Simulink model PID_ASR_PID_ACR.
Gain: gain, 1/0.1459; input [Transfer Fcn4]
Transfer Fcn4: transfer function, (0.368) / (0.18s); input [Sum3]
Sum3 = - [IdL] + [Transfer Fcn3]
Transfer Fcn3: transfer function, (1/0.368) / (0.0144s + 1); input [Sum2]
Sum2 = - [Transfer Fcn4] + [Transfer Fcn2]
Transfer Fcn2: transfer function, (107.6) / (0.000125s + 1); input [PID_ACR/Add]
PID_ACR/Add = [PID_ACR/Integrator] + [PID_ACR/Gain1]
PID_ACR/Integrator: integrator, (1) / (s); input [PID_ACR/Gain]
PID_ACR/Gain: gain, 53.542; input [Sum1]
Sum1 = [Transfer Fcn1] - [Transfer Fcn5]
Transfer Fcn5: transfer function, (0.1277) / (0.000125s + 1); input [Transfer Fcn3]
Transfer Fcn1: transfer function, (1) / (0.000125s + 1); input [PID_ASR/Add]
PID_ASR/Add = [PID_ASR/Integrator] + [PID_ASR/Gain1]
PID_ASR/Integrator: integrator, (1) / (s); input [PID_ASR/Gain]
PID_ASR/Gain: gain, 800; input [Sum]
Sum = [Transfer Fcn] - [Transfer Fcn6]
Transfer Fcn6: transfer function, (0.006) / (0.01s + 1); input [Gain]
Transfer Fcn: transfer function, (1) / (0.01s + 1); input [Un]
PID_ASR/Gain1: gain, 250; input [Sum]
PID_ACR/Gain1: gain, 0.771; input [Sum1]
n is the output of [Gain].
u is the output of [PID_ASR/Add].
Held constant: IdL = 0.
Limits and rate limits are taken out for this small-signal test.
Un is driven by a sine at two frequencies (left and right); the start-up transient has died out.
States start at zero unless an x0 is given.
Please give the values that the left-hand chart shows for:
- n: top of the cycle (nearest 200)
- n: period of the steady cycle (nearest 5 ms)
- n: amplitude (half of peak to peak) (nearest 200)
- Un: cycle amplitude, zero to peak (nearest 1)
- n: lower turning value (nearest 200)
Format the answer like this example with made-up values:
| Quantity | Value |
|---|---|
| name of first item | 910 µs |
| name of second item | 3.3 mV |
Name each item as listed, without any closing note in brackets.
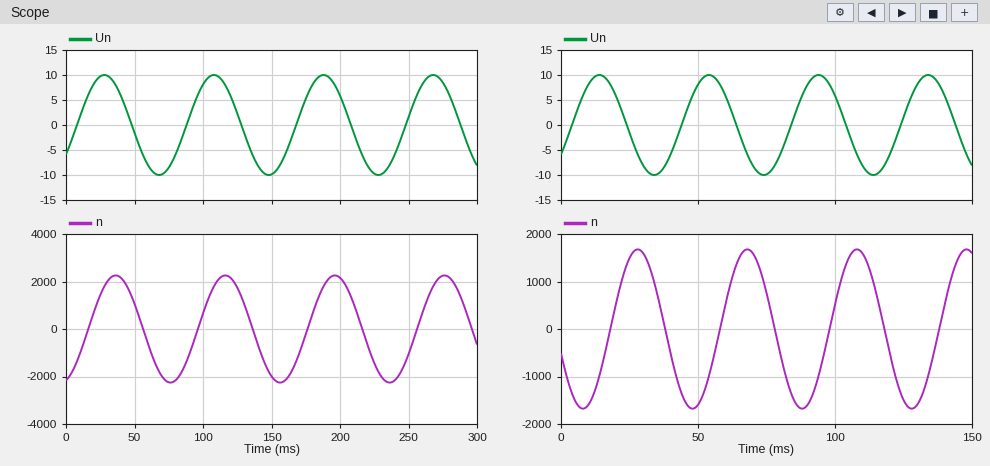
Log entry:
| Quantity | Value |
|---|---|
| n: top of the cycle | 2200 |
| n: period of the steady cycle | 80 ms |
| n: amplitude (half of peak to peak) | 2200 |
| Un: cycle amplitude, zero to peak | 10 |
| n: lower turning value | -2200 |
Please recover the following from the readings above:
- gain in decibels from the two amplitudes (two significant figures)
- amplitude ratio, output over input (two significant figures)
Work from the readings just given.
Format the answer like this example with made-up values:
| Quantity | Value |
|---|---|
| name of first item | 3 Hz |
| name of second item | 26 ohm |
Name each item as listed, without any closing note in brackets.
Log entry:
| Quantity | Value |
|---|---|
| gain in decibels from the two amplitudes | 47 dB |
| amplitude ratio, output over input | 220 |
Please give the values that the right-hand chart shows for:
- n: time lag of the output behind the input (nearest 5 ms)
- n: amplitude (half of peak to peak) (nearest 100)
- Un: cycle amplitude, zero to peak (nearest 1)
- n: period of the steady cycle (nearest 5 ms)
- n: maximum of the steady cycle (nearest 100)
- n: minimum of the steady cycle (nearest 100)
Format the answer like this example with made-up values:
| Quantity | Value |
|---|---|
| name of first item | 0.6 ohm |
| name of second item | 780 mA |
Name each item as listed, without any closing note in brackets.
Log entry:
| Quantity | Value |
|---|---|
| n: time lag of the output behind the input | 15 ms |
| n: amplitude (half of peak to peak) | 1700 |
| Un: cycle amplitude, zero to peak | 10 |
| n: period of the steady cycle | 40 ms |
| n: maximum of the steady cycle | 1700 |
| n: minimum of the steady cycle | -1700 |
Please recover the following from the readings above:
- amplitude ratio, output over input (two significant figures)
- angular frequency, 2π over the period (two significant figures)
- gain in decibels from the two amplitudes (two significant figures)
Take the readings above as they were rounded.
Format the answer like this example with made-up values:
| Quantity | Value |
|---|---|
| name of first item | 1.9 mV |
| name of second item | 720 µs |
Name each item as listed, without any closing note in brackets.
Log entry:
| Quantity | Value |
|---|---|
| amplitude ratio, output over input | 170 |
| angular frequency, 2π over the period | 0.16 rad/ms |
| gain in decibels from the two amplitudes | 45 dB |
